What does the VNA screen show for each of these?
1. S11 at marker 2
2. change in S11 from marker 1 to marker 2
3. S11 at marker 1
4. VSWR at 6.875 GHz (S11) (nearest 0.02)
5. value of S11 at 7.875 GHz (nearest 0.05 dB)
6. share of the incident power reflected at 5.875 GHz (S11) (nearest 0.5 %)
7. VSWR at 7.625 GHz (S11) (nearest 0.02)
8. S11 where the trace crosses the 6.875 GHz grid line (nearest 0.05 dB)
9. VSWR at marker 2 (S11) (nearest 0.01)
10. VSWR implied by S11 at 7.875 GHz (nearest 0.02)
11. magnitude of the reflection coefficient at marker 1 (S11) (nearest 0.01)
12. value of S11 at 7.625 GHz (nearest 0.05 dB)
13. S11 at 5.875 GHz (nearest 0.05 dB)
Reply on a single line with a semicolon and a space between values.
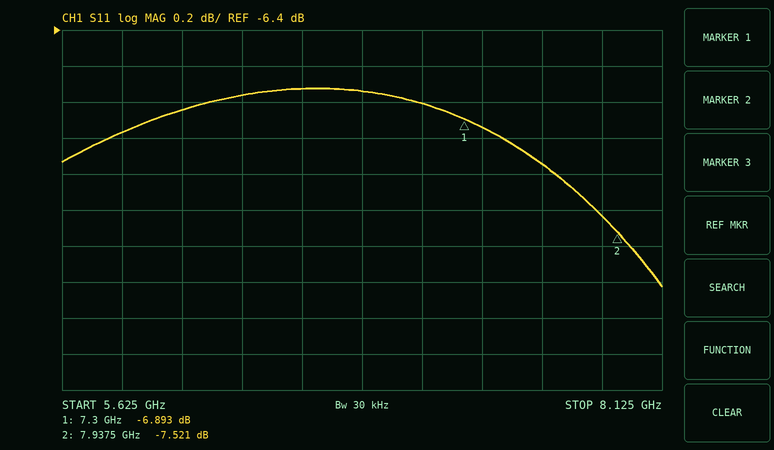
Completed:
-7.521 dB; -0.628 dB; -6.893 dB; 2.70; -7.45 dB; 20.0 %; 2.56; -6.75 dB; 2.45; 2.48; 0.45; -7.15 dB; -6.95 dB
